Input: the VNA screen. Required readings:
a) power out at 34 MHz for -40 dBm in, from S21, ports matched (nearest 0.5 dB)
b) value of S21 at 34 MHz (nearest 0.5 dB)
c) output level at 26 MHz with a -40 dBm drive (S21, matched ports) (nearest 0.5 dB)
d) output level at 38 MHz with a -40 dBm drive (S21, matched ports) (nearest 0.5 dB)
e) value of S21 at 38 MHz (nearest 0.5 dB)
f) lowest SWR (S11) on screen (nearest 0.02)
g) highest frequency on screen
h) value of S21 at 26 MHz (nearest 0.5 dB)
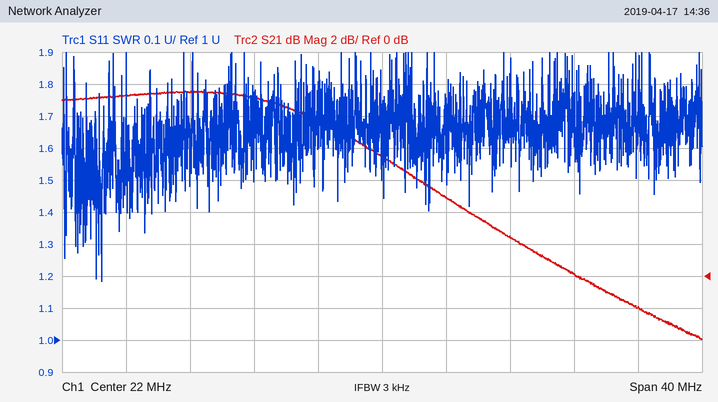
-40.0 dBm
0.0 dB
-35.0 dBm
-42.0 dBm
-2.0 dB
1.18
42 MHz
5.0 dB
